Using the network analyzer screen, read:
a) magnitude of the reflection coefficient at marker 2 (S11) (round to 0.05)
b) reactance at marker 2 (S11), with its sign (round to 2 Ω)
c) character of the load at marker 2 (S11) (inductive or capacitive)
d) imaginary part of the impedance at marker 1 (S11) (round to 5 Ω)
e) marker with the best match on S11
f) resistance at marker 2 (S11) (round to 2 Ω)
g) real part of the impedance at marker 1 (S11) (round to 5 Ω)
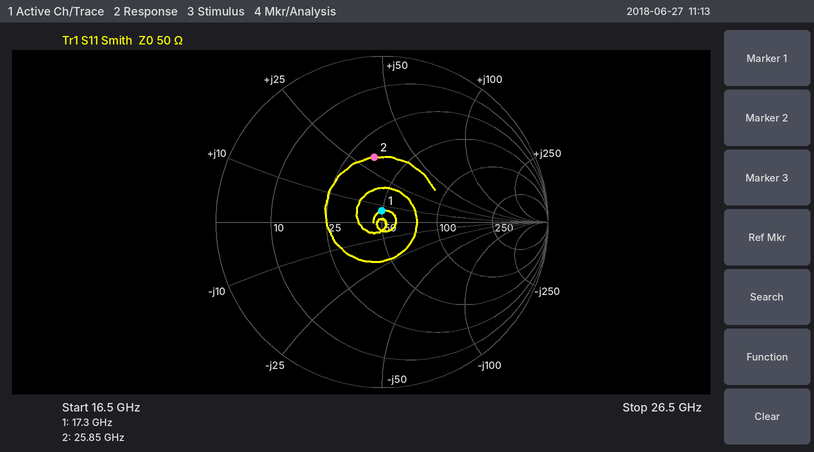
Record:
0.40
+32 Ω
inductive
+5 Ω
marker 1
34 Ω
50 Ω
